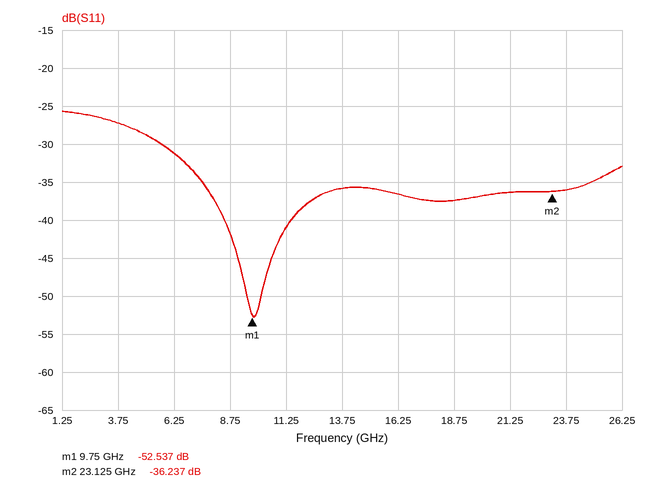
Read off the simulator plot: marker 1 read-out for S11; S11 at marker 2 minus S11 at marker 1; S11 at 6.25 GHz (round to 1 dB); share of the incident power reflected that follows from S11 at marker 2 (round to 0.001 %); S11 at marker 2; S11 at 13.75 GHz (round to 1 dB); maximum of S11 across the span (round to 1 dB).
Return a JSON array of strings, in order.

["-52.537 dB", "16.300 dB", "-31 dB", "0.024 %", "-36.237 dB", "-36 dB", "-26 dB"]
